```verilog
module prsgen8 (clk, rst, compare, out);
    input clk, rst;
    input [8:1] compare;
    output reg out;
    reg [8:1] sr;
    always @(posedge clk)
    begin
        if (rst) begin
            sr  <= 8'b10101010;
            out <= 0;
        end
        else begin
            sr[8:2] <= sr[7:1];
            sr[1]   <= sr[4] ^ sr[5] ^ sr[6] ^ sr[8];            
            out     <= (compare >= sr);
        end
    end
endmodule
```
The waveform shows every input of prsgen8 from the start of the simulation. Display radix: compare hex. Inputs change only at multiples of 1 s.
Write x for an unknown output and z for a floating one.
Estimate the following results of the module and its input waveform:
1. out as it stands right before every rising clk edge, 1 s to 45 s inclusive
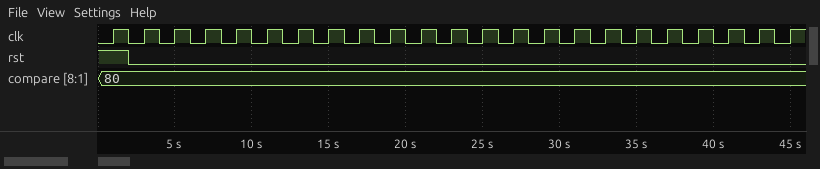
x 0 0 1 0 1 0 1 0 1 0 0 0 0 0 1 1 0 1 0 1 1 1
